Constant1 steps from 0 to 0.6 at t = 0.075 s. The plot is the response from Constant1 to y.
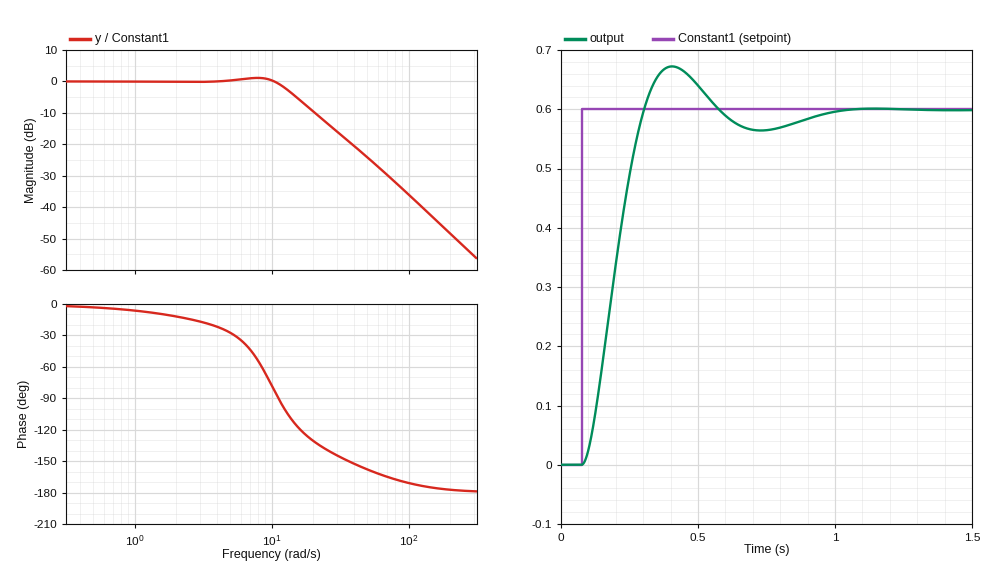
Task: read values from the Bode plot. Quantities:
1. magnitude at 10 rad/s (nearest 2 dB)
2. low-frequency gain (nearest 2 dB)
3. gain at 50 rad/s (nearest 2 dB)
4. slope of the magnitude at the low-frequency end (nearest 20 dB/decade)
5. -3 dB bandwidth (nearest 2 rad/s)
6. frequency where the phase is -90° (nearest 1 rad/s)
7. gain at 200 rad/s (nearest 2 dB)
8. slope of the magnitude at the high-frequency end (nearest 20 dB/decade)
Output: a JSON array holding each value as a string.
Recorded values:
["0 dB", "0 dB", "-24 dB", "0 dB/decade", "14 rad/s", "11 rad/s", "-48 dB", "-40 dB/decade"]
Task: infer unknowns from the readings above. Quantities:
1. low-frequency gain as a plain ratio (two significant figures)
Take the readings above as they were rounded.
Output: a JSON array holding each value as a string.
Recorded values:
["1.0"]
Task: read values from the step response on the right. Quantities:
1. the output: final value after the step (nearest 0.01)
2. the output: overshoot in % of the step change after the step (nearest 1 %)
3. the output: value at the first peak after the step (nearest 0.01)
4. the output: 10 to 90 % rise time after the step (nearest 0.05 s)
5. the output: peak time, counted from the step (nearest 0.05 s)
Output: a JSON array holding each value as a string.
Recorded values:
["0.60", "12 %", "0.67", "0.15 s", "0.35 s"]
